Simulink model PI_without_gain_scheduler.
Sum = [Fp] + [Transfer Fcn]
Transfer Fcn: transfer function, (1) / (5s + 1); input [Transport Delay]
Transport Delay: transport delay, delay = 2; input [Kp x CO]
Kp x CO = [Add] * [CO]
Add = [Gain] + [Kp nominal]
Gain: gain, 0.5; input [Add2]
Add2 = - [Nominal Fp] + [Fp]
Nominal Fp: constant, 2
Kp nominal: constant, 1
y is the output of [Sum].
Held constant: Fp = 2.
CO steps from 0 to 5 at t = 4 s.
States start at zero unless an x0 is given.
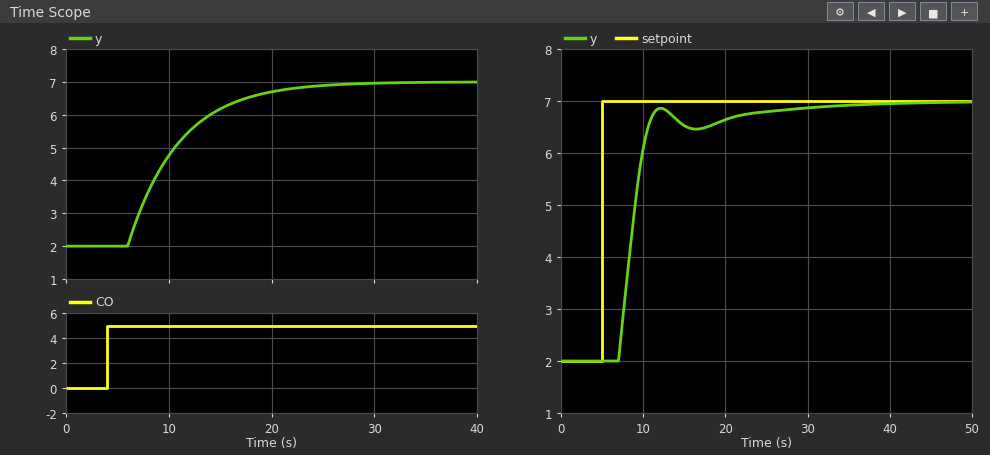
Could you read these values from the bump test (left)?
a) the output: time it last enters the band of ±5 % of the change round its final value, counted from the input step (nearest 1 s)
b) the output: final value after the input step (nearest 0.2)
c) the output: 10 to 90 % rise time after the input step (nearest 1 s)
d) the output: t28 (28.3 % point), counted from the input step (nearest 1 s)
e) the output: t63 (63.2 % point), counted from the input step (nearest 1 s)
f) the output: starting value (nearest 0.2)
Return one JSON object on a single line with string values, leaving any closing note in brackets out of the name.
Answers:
{"the output: time it last enters the band of ±5 % of the change round its final value, counted from the input step": "17 s", "the output: final value after the input step": "7.0", "the output: 10 to 90 % rise time after the input step": "11 s", "the output: t28 (28.3 % point), counted from the input step": "4 s", "the output: t63 (63.2 % point), counted from the input step": "7 s", "the output: starting value": "2.0"}
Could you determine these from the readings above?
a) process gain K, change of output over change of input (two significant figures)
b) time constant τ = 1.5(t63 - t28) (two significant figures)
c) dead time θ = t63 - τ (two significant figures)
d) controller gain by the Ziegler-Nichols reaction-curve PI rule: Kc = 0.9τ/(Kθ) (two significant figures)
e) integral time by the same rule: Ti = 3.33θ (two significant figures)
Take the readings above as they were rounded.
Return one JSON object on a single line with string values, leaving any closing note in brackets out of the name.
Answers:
{"process gain K, change of output over change of input": "1.0", "time constant τ = 1.5(t63 - t28)": "4.5 s", "dead time θ = t63 - τ": "2.5 s", "controller gain by the Ziegler-Nichols reaction-curve PI rule: Kc = 0.9τ/(Kθ)": "1.6", "integral time by the same rule: Ti = 3.33θ": "8.3 s"}
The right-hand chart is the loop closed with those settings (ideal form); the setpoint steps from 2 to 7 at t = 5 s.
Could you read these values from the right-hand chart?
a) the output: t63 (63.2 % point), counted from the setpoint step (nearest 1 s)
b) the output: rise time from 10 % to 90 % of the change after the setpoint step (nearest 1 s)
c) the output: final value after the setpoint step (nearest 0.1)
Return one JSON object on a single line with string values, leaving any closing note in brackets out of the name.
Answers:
{"the output: t63 (63.2 % point), counted from the setpoint step": "4 s", "the output: rise time from 10 % to 90 % of the change after the setpoint step": "3 s", "the output: final value after the setpoint step": "7.0"}
